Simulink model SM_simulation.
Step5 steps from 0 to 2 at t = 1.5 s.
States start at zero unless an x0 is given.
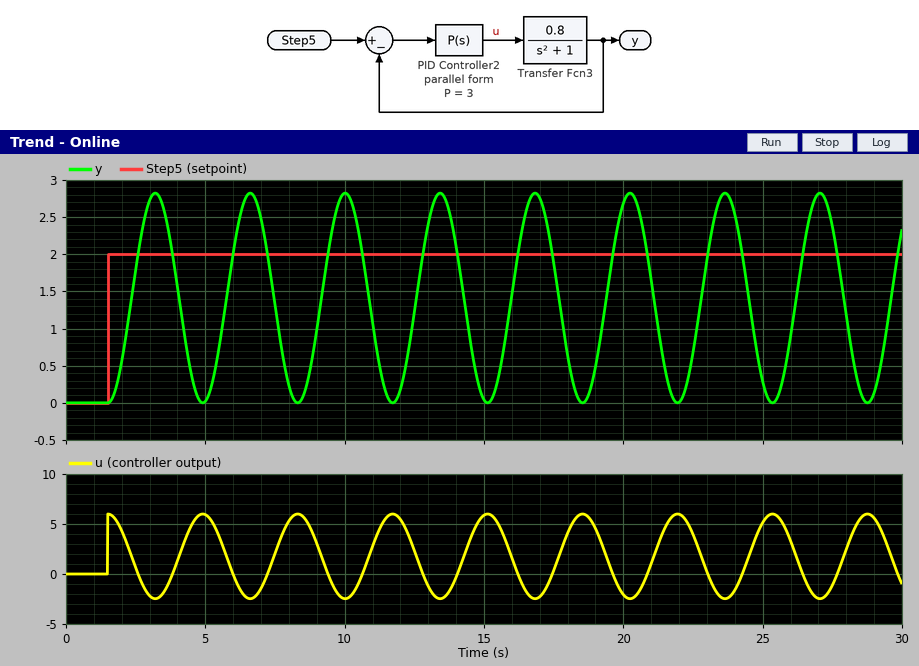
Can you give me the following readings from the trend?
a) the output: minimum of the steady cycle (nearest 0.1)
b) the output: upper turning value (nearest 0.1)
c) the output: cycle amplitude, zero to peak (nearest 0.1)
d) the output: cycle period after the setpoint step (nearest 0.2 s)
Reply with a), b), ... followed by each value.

a) 0.0
b) 2.8
c) 1.4
d) 3.4 s
